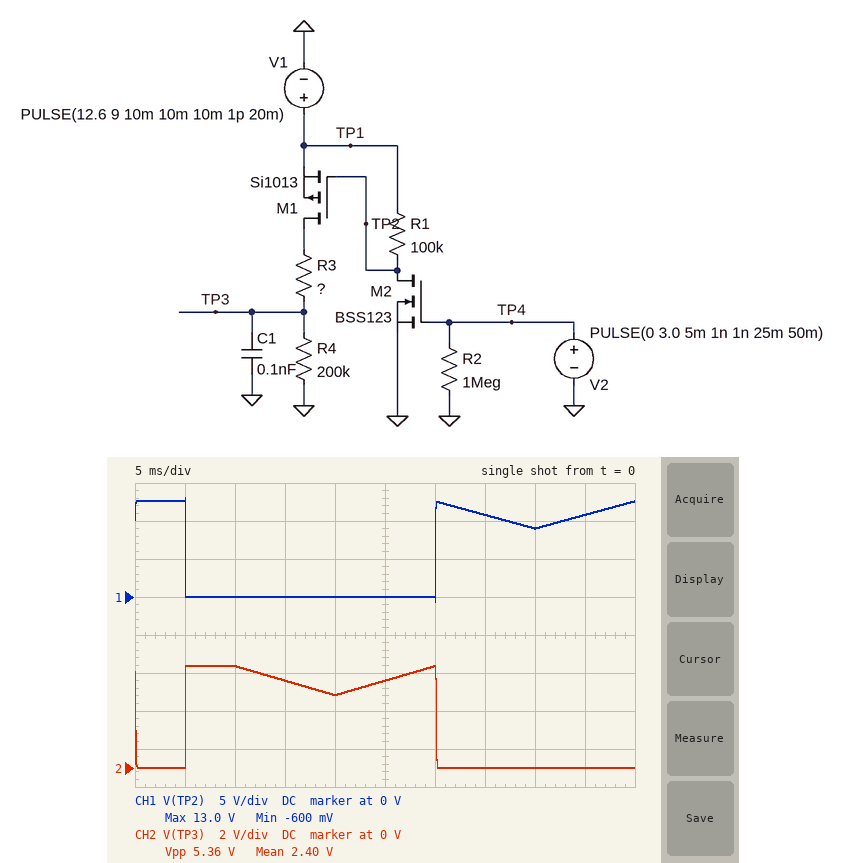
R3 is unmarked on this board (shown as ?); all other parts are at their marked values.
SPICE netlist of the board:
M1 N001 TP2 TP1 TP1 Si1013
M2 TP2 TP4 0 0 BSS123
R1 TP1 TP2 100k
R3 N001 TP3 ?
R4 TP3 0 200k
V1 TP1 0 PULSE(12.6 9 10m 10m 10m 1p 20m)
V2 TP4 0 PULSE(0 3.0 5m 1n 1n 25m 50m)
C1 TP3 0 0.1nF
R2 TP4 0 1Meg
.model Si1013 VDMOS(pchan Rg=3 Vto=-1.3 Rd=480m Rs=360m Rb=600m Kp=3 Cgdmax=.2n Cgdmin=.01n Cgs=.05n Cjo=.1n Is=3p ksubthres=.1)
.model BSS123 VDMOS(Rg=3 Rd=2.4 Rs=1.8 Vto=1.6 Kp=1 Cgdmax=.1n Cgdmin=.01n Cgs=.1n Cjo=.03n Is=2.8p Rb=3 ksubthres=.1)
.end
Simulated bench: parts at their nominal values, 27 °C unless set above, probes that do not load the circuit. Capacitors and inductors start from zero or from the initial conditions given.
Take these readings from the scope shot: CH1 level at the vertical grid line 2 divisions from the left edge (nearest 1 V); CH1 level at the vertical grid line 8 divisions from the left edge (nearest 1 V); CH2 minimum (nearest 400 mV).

0 V
9 V
0 V
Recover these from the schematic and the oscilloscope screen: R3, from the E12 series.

270 kΩ
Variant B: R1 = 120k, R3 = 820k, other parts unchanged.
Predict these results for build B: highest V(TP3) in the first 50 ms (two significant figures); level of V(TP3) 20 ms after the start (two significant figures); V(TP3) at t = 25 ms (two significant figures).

2.5 V
1.8 V
2.1 V
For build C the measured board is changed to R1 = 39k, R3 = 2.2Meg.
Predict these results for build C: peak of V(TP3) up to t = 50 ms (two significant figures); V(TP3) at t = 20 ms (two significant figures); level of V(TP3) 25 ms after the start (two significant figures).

1.1 V
750 mV
900 mV
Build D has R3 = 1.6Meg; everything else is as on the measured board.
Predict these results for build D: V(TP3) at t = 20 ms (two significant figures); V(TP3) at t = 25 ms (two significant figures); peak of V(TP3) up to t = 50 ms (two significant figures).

1.0 V
1.2 V
1.4 V
